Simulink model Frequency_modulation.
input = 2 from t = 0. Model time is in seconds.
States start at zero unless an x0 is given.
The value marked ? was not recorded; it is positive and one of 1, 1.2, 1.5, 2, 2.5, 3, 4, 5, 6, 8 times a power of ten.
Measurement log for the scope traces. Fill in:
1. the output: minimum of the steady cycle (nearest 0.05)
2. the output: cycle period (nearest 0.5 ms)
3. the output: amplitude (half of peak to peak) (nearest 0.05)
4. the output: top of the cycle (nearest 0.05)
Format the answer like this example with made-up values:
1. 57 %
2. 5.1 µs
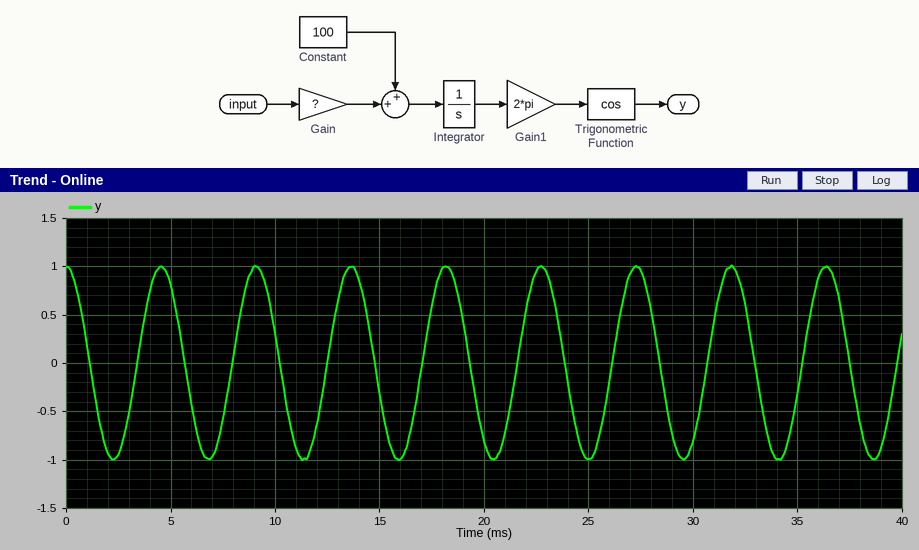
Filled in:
1. -1.00
2. 4.5 ms
3. 1.00
4. 1.00
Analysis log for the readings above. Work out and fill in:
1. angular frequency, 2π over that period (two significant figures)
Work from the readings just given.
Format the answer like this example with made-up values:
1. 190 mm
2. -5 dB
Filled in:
1. 1.4 rad/ms
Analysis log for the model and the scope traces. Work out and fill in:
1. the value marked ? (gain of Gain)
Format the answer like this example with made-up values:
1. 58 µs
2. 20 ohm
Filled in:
1. 60
